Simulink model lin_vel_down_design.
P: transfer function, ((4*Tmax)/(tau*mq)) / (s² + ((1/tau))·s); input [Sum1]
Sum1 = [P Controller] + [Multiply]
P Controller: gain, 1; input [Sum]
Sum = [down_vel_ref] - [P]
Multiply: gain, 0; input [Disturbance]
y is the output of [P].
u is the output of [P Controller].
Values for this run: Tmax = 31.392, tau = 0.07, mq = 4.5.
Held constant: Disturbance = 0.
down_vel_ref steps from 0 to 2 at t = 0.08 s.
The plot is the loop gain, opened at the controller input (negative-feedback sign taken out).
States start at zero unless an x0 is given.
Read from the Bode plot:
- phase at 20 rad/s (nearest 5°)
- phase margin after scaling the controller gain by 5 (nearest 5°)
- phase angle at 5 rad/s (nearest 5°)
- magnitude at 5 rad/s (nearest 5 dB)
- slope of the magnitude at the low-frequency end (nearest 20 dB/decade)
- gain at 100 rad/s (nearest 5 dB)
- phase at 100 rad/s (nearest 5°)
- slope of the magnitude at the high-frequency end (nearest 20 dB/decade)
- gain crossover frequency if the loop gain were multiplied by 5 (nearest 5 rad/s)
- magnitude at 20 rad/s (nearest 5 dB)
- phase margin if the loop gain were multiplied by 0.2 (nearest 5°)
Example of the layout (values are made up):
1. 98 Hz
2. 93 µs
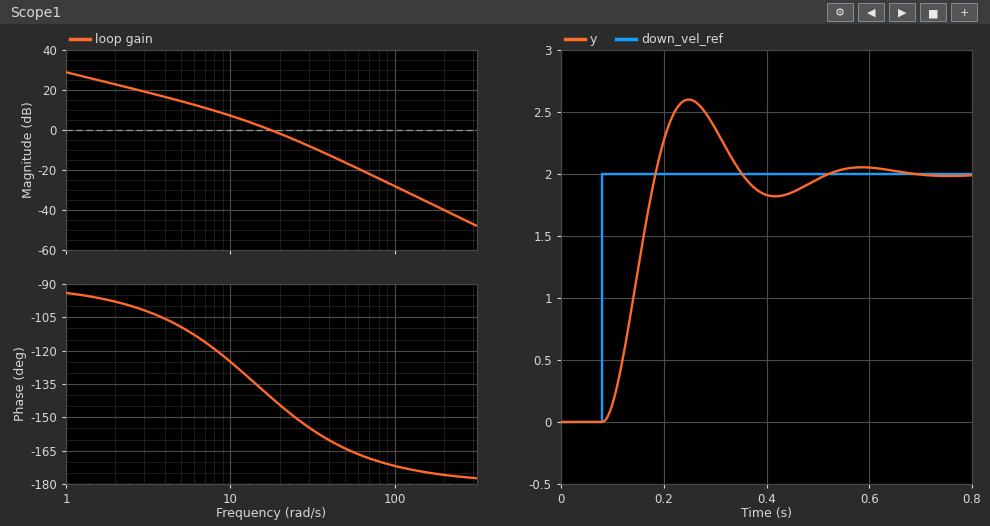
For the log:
1. -145°
2. 20°
3. -110°
4. 15 dB
5. -20 dB/decade
6. -30 dB
7. -170°
8. -40 dB/decade
9. 45 rad/s
10. 0 dB
11. 70°
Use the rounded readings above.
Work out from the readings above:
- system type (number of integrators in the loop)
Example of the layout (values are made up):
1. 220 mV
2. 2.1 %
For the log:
1. 1
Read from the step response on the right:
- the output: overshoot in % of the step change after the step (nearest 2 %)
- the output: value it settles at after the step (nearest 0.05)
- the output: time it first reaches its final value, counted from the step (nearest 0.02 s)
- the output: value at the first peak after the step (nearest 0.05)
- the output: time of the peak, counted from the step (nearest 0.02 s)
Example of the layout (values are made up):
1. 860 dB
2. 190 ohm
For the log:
1. 30 %
2. 2.00
3. 0.10 s
4. 2.60
5. 0.16 s
